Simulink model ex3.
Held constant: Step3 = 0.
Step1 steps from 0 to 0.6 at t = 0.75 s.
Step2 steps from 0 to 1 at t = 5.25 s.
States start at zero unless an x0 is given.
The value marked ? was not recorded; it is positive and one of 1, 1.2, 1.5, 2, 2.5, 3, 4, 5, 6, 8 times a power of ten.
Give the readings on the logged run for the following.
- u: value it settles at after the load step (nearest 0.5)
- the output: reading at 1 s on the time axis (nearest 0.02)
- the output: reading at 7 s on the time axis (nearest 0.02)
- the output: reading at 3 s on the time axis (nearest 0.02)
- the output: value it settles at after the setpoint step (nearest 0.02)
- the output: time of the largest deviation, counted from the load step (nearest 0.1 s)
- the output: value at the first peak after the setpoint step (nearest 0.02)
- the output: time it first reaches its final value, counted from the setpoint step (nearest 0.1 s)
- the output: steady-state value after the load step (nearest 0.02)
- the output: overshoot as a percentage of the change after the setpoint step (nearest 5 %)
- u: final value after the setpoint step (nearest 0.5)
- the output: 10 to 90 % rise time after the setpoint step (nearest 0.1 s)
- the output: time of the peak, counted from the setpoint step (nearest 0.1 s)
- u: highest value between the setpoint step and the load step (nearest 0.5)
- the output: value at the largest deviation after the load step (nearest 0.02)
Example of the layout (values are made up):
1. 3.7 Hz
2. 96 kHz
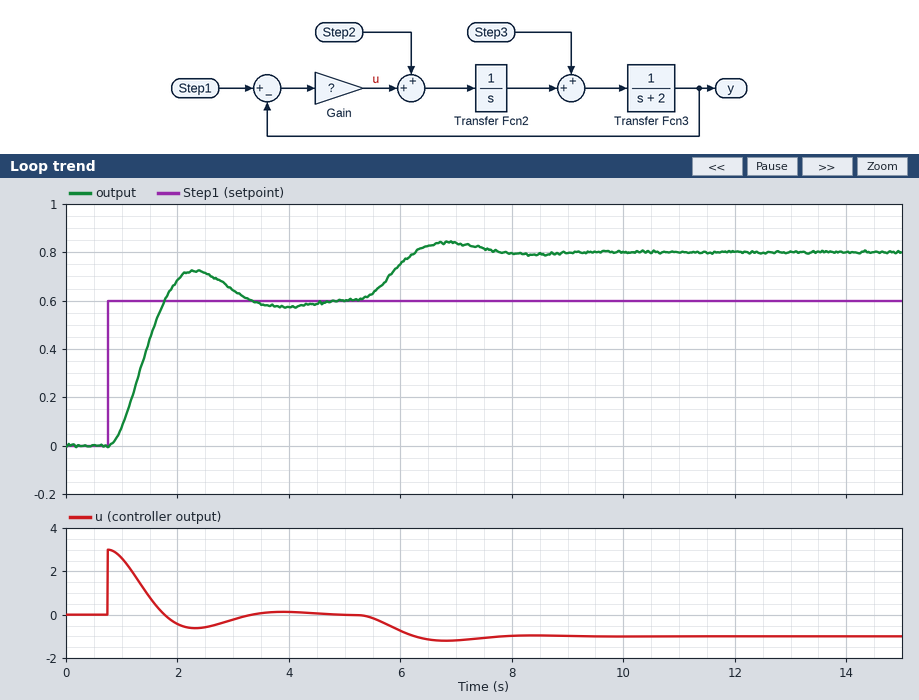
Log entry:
1. -1.0
2. 0.08
3. 0.84
4. 0.64
5. 0.60
6. 1.6 s
7. 0.72
8. 1.0 s
9. 0.80
10. 20 %
11. 0.0
12. 0.7 s
13. 1.6 s
14. 3.0
15. 0.84
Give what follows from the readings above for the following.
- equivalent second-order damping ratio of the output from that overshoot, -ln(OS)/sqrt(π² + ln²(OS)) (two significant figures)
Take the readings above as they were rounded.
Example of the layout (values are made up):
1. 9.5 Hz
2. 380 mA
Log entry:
1. 0.46
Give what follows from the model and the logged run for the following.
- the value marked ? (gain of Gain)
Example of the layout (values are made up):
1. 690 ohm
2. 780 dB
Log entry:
1. 5
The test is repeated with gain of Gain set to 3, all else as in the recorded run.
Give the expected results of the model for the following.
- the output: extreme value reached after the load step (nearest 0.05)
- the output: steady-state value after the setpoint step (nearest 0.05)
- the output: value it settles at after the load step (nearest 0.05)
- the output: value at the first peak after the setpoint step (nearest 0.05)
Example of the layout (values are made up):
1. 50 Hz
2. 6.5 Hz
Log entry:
1. 0.95
2. 0.60
3. 0.95
4. 0.65
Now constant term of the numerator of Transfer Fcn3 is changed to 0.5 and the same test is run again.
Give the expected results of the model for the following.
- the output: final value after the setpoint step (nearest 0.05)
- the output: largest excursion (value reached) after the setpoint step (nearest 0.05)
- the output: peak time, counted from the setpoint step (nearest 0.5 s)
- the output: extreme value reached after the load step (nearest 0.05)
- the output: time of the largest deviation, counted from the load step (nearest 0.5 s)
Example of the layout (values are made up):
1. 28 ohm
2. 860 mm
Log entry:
1. 0.60
2. 0.65
3. 2.5 s
4. 0.80
5. 2.5 s
